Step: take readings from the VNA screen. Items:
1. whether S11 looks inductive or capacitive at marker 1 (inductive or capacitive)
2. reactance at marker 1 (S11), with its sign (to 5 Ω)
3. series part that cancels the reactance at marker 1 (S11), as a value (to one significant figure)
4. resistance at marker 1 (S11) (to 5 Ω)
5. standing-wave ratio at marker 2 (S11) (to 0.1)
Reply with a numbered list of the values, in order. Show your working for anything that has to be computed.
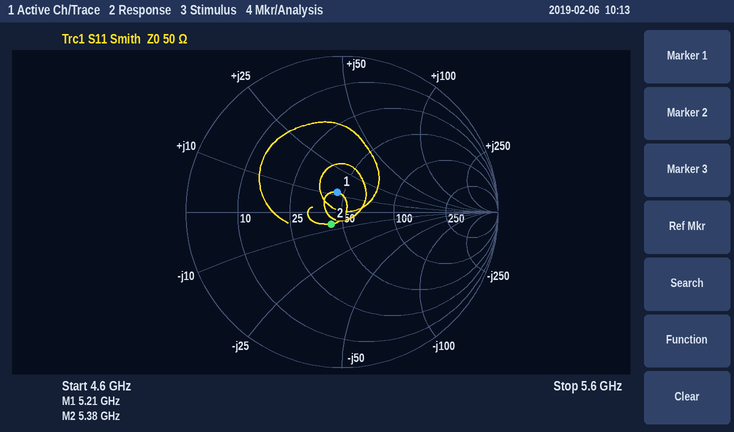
1. inductive
2. +10 Ω
3. C = 1/(2π × 5.21 GHz × 10 Ω) ≈ 3 pF
4. 45 Ω
5. 1.2
